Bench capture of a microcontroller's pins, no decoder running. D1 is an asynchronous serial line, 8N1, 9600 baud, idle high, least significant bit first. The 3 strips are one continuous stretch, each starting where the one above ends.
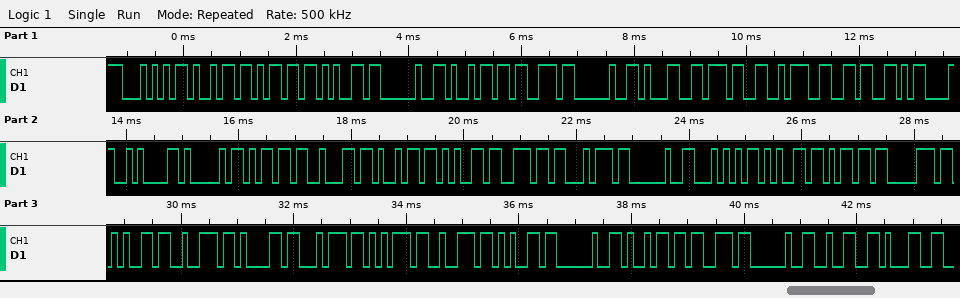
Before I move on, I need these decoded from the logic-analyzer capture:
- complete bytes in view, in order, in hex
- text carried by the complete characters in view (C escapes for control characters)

54 69 6D 65 20 69 73 20 31 37 3A 36 0D 0A 41 6D 62 69 65 6E 74 20 54 65 6D 70 65 72 61 74 75 72 65 20 69 73 20 32 31
"Time is 17:6\r\nAmbient Temperature is 21"
